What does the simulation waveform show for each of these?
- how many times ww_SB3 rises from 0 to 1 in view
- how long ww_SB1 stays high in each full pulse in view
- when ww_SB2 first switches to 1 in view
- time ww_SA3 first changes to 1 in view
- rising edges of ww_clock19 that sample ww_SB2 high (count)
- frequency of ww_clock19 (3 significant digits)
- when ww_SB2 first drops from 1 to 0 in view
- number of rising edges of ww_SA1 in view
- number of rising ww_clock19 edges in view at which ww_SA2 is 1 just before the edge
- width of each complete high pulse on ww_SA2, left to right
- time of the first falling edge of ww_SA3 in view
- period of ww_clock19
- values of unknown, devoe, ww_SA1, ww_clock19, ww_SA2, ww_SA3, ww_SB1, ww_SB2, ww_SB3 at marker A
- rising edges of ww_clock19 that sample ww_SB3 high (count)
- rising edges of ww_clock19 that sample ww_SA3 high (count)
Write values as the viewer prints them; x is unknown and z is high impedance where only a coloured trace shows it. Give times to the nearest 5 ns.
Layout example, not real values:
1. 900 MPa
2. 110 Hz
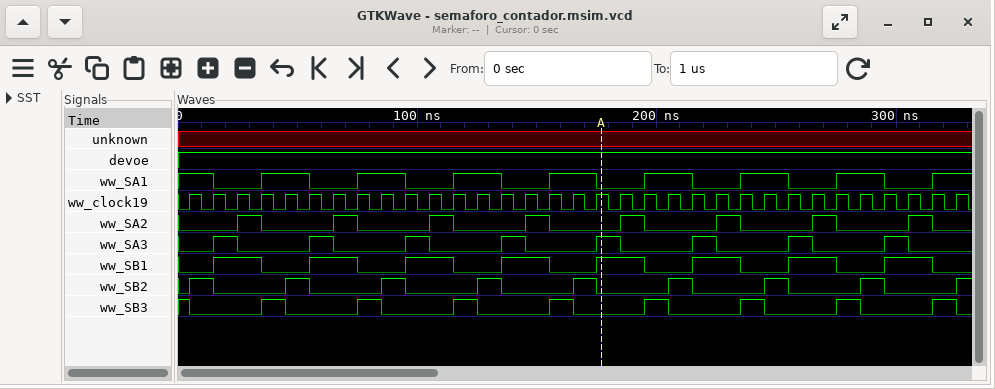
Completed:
1. 8
2. 20 ns, 20 ns, 20 ns, 20 ns, 20 ns, 20 ns, 20 ns, 20 ns
3. 5 ns
4. 15 ns
5. 8
6. 100 MHz
7. 15 ns
8. 8
9. 8
10. 10 ns, 10 ns, 10 ns, 10 ns, 10 ns, 10 ns, 10 ns, 10 ns
11. 25 ns
12. 10 ns
13. unknown=x, devoe=1, ww_SA1=0, ww_clock19=1, ww_SA2=0, ww_SA3=1, ww_SB1=1, ww_SB2=0, ww_SB3=0
14. 9
15. 8
